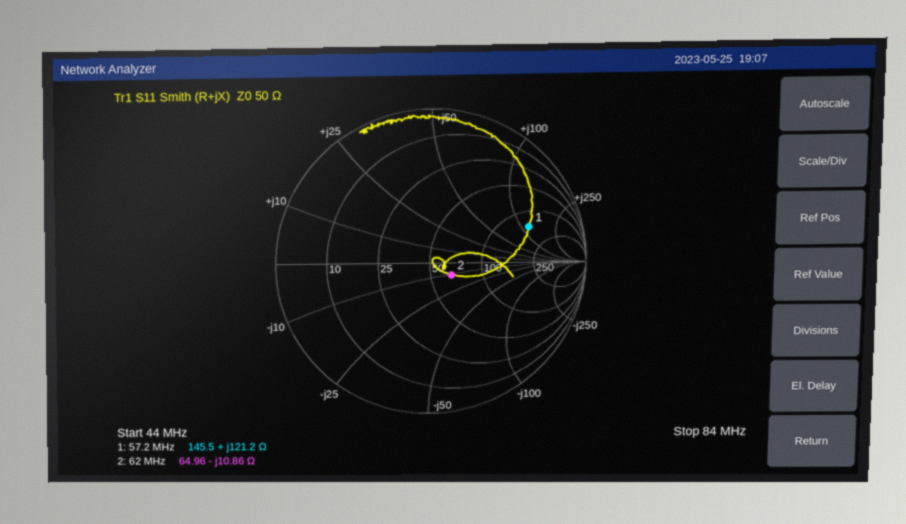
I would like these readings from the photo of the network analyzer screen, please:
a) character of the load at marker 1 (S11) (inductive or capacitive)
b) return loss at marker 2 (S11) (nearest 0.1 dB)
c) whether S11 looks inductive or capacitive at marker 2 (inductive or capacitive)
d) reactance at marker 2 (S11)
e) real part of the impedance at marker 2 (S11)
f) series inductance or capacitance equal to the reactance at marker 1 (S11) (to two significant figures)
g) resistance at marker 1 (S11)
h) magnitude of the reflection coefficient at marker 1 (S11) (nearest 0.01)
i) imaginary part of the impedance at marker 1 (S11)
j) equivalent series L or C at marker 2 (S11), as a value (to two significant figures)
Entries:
inductive
15.9 dB
capacitive
-10.86 Ω
64.96 Ω
340 nH
145.5 Ω
0.67
+121.2 Ω
240 pF
